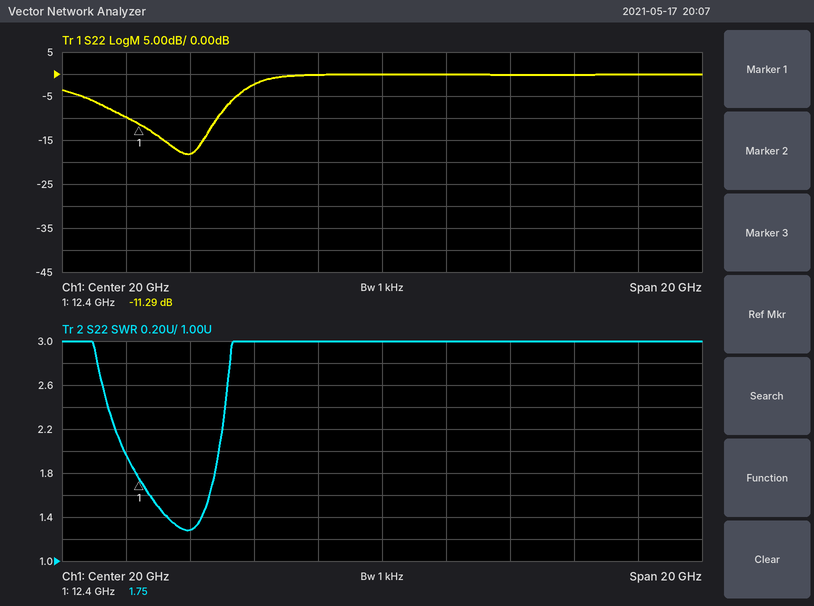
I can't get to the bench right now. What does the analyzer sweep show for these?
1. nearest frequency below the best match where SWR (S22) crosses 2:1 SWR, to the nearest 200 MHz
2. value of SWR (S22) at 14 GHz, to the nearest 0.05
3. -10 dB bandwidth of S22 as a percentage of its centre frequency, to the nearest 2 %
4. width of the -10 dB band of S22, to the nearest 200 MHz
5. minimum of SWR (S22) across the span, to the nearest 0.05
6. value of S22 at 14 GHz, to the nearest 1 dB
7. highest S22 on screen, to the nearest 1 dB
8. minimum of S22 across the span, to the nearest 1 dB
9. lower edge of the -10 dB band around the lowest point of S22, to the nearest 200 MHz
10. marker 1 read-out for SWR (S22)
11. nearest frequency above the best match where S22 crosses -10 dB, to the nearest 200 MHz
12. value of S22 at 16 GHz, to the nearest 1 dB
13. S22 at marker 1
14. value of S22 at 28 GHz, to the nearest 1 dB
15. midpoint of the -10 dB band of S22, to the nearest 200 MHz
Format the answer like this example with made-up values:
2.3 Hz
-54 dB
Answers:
12.0 GHz
1.30
20 %
2.8 GHz
1.30
-18 dB
0 dB
-18 dB
12.0 GHz
1.75
14.8 GHz
-2 dB
-11.29 dB
0 dB
13.4 GHz
